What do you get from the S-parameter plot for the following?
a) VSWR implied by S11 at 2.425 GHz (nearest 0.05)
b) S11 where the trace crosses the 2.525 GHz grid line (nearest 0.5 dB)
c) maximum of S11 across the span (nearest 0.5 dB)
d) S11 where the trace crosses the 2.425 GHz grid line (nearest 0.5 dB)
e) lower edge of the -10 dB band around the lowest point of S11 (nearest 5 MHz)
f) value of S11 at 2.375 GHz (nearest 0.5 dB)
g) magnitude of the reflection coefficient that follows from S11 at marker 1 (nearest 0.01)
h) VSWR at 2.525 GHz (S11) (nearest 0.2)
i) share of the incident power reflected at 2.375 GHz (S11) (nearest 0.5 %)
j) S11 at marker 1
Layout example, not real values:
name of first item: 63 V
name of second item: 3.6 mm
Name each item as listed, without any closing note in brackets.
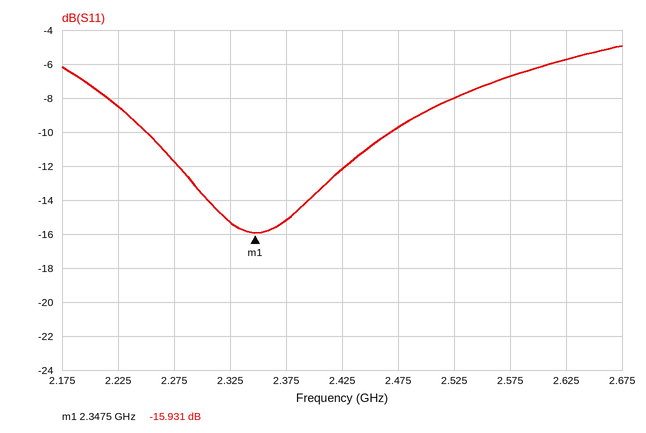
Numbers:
VSWR implied by S11 at 2.425 GHz: 1.65
S11 where the trace crosses the 2.525 GHz grid line: -8.0 dB
maximum of S11 across the span: -5.0 dB
S11 where the trace crosses the 2.425 GHz grid line: -12.0 dB
lower edge of the -10 dB band around the lowest point of S11: 2.250 GHz
value of S11 at 2.375 GHz: -15.0 dB
magnitude of the reflection coefficient that follows from S11 at marker 1: 0.16
VSWR at 2.525 GHz (S11): 2.4
share of the incident power reflected at 2.375 GHz (S11): 3.0 %
S11 at marker 1: -15.931 dB
